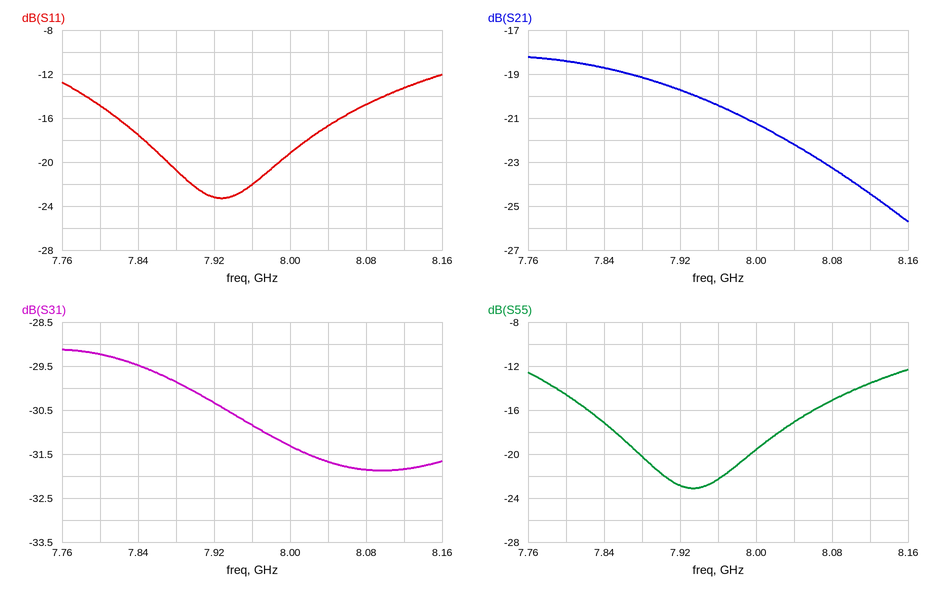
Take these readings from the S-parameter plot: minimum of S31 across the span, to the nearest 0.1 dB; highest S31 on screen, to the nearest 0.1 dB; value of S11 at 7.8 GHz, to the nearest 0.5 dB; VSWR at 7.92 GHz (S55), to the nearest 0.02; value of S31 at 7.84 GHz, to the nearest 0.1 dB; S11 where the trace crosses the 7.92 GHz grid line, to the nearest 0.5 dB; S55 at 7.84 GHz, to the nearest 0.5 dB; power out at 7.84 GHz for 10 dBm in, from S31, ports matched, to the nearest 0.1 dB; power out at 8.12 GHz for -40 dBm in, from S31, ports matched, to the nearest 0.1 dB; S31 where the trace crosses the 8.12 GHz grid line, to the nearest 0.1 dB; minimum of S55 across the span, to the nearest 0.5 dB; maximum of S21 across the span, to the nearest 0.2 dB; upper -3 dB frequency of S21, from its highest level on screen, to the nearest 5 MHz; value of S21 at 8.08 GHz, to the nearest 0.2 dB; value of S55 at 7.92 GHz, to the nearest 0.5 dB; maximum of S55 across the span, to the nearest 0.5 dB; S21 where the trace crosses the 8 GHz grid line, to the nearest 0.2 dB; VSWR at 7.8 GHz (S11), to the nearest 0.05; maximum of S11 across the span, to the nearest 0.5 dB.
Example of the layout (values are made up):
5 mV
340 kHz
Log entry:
-31.9 dB
-29.1 dB
-15.0 dB
1.16
-29.5 dB
-23.0 dB
-17.0 dB
-19.5 dBm
-71.8 dBm
-31.8 dB
-23.0 dB
-18.2 dB
8.000 GHz
-23.2 dB
-23.0 dB
-12.5 dB
-21.2 dB
1.45
-12.0 dB
